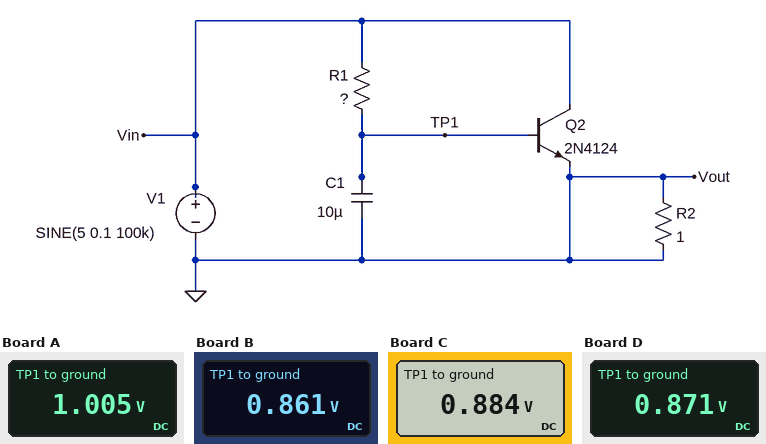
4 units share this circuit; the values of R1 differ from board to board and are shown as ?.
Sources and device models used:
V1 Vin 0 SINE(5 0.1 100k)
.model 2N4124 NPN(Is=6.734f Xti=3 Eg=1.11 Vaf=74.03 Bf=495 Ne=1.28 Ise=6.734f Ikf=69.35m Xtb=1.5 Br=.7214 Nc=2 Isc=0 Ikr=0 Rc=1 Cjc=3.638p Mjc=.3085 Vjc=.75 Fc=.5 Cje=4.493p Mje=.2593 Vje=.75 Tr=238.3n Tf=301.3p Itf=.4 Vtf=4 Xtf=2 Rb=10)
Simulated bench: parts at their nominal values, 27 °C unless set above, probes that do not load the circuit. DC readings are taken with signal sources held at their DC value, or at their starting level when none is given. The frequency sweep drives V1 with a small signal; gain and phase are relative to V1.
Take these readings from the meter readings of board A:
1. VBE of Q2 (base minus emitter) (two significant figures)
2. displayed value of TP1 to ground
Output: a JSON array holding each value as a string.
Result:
["1.0 V", "1.005 V"]
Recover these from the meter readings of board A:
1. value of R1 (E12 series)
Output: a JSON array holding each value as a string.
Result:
["330 Ω"]
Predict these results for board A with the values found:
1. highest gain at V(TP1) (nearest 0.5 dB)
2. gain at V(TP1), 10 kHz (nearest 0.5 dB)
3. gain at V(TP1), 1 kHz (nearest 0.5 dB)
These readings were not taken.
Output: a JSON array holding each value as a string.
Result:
["-29.0 dB", "-46.5 dB", "-31.0 dB"]
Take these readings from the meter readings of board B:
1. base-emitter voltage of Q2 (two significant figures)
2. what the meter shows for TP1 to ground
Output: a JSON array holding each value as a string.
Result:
["860 mV", "0.861 V"]
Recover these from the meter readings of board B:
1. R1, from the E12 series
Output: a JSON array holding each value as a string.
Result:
["1.8 kΩ"]
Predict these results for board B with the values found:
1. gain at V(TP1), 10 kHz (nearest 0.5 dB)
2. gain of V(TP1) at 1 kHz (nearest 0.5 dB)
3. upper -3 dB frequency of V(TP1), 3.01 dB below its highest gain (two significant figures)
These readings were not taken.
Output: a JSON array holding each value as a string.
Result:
["-61.0 dB", "-43.0 dB", "730 Hz"]
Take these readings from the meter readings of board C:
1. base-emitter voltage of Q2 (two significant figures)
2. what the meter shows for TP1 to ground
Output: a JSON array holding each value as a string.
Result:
["880 mV", "0.884 V"]
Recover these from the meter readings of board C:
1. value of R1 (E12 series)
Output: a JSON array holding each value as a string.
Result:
["1.2 kΩ"]
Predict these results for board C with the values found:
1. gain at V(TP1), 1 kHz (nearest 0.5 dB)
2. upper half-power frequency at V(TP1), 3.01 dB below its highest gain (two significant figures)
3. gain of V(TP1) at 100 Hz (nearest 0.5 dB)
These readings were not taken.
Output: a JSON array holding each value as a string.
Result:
["-40.0 dB", "900 Hz", "-36.5 dB"]
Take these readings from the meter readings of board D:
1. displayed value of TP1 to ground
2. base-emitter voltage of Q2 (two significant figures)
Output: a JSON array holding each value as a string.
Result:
["0.871 V", "870 mV"]
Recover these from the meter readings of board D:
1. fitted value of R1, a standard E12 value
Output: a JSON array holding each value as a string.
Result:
["1.5 kΩ"]
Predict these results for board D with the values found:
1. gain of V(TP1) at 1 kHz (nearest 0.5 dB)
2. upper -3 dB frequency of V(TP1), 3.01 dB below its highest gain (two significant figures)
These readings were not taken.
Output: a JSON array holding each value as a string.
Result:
["-41.5 dB", "810 Hz"]
